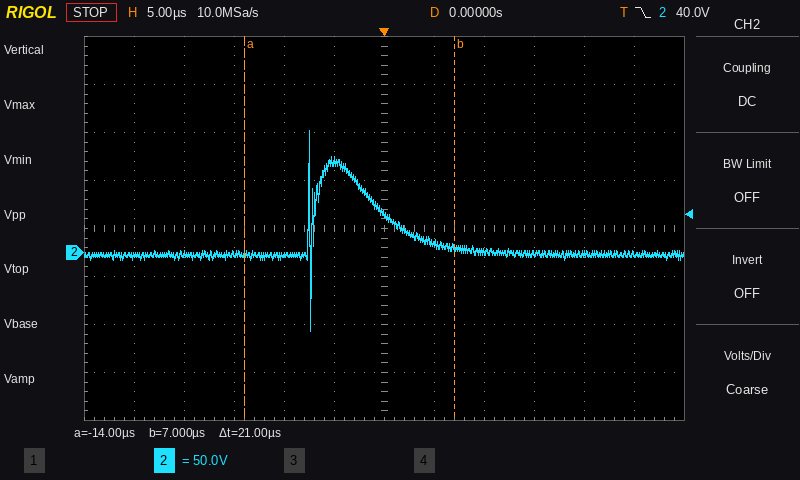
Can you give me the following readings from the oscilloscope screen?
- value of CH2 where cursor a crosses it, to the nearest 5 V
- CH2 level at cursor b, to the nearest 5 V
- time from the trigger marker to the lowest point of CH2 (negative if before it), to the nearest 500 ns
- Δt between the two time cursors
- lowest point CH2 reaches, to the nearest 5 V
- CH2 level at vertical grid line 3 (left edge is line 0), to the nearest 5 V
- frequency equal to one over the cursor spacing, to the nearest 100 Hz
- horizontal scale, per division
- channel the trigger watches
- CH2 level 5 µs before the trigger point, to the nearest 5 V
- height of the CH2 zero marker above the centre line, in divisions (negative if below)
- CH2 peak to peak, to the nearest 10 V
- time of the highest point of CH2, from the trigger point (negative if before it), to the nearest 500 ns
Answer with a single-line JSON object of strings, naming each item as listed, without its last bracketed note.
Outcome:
{"value of CH2 where cursor a crosses it, to the nearest 5 V": "0 V", "CH2 level at cursor b, to the nearest 5 V": "5 V", "time from the trigger marker to the lowest point of CH2 (negative if before it), to the nearest 500 ns": "-7.5 µs", "Δt between the two time cursors": "21 µs", "lowest point CH2 reaches, to the nearest 5 V": "-80 V", "CH2 level at vertical grid line 3 (left edge is line 0), to the nearest 5 V": "0 V", "frequency equal to one over the cursor spacing, to the nearest 100 Hz": "47.6 kHz", "horizontal scale, per division": "5 µs", "channel the trigger watches": "CH2", "CH2 level 5 µs before the trigger point, to the nearest 5 V": "95 V", "height of the CH2 zero marker above the centre line, in divisions": "-0.5 div", "CH2 peak to peak, to the nearest 10 V": "210 V", "time of the highest point of CH2, from the trigger point (negative if before it), to the nearest 500 ns": "-7.5 µs"}
